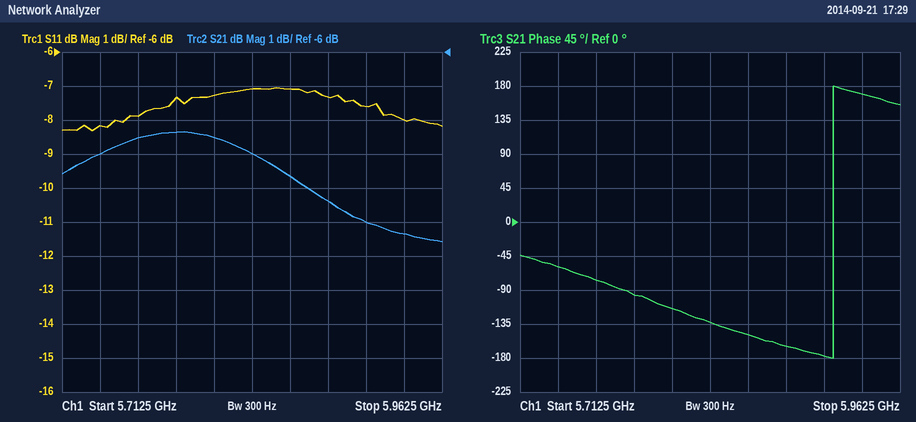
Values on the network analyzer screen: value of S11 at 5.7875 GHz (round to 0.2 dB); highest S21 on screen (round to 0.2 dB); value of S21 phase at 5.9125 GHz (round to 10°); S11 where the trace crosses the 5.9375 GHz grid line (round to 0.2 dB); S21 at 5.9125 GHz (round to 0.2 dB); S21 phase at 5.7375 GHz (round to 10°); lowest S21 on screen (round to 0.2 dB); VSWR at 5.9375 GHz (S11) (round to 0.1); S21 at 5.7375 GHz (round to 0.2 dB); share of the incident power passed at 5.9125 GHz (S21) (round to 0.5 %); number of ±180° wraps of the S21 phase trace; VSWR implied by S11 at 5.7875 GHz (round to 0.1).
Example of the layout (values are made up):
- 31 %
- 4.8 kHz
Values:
- -7.4 dB
- -8.4 dB
- -180°
- -8.0 dB
- -11.0 dB
- -60°
- -11.6 dB
- 2.3
- -9.0 dB
- 8.0 %
- 1
- 2.5
